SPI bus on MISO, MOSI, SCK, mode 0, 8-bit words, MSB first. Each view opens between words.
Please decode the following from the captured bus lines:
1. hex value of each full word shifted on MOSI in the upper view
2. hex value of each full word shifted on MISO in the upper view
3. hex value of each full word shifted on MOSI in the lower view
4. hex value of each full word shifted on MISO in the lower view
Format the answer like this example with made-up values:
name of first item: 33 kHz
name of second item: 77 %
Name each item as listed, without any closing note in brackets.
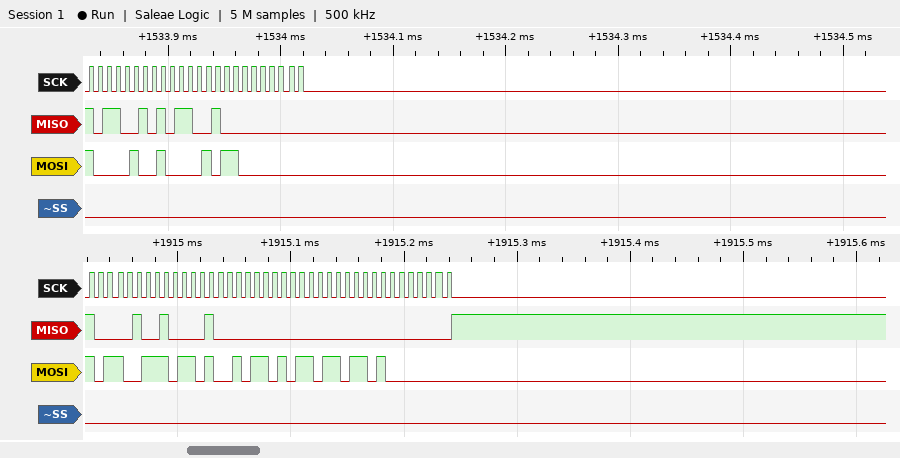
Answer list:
hex value of each full word shifted on MOSI in the upper view: 84, 85, 80
hex value of each full word shifted on MISO in the upper view: B2, B2, 00
hex value of each full word shifted on MOSI in the lower view: B3, B4, B5, B6, 80
hex value of each full word shifted on MISO in the lower view: 84, 84, 00, 00, 00
